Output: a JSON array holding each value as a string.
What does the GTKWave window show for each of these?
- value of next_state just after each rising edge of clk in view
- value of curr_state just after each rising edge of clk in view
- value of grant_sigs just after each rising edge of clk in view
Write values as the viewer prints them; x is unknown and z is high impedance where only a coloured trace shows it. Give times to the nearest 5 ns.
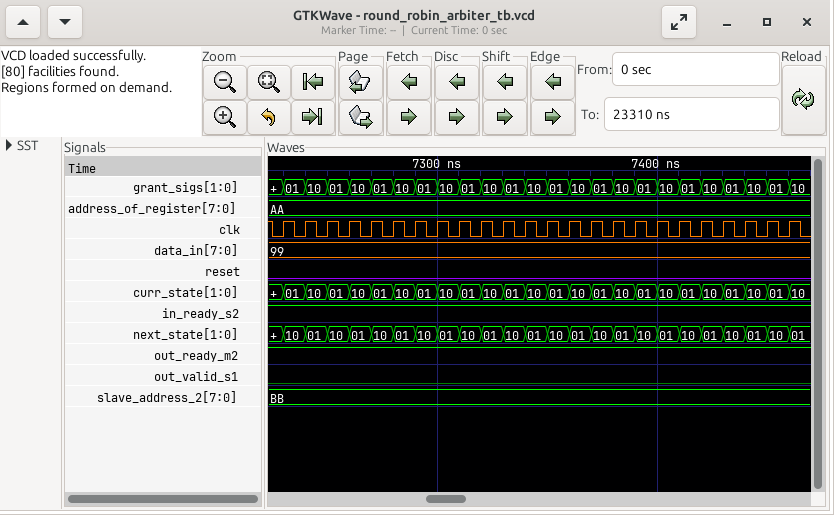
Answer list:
["10, 01, 10, 01, 10, 01, 10, 01, 10, 01, 10, 01, 10, 01, 10, 01, 10, 01, 10, 01, 10, 01, 10, 01", "01, 10, 01, 10, 01, 10, 01, 10, 01, 10, 01, 10, 01, 10, 01, 10, 01, 10, 01, 10, 01, 10, 01, 10", "01, 10, 01, 10, 01, 10, 01, 10, 01, 10, 01, 10, 01, 10, 01, 10, 01, 10, 01, 10, 01, 10, 01, 10"]
